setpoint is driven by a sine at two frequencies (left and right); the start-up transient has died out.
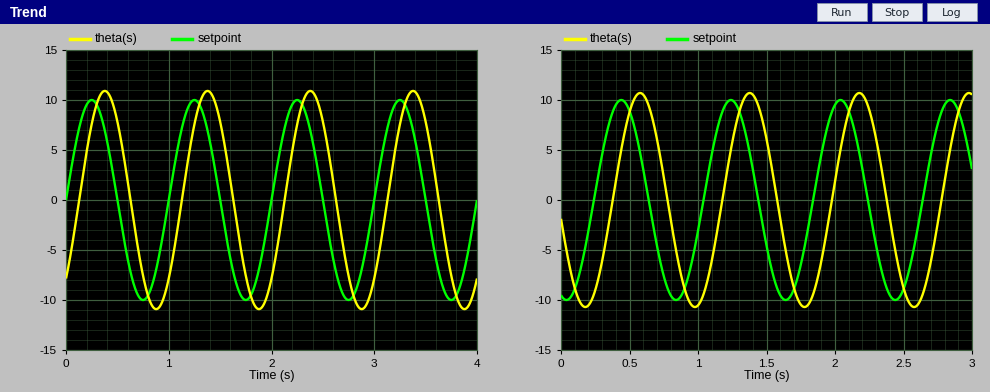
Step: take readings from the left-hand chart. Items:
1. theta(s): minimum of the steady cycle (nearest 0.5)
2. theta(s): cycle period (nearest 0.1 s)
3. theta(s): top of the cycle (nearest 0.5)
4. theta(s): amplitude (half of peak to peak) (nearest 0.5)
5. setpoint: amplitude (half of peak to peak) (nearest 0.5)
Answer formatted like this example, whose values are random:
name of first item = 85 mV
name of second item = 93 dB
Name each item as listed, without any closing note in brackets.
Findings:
theta(s): minimum of the steady cycle = -11.0
theta(s): cycle period = 1.0 s
theta(s): top of the cycle = 11.0
theta(s): amplitude (half of peak to peak) = 11.0
setpoint: amplitude (half of peak to peak) = 10.0
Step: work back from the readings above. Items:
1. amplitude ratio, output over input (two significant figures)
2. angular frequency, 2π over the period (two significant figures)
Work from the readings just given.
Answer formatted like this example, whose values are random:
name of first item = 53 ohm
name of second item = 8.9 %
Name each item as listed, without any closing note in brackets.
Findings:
amplitude ratio, output over input = 1.1
angular frequency, 2π over the period = 6.3 rad/s
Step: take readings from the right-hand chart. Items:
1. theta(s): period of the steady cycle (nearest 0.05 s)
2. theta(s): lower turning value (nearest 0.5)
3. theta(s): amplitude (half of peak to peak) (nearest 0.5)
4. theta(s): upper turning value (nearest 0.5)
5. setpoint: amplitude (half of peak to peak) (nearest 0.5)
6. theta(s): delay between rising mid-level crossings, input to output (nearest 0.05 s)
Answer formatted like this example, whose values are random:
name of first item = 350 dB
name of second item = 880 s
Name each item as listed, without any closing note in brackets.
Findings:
theta(s): period of the steady cycle = 0.80 s
theta(s): lower turning value = -10.5
theta(s): amplitude (half of peak to peak) = 10.5
theta(s): upper turning value = 10.5
setpoint: amplitude (half of peak to peak) = 10.0
theta(s): delay between rising mid-level crossings, input to output = 0.15 s
